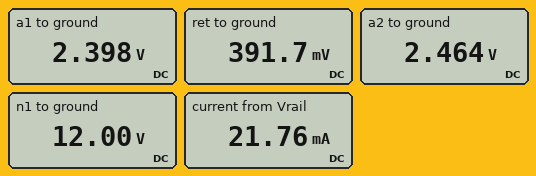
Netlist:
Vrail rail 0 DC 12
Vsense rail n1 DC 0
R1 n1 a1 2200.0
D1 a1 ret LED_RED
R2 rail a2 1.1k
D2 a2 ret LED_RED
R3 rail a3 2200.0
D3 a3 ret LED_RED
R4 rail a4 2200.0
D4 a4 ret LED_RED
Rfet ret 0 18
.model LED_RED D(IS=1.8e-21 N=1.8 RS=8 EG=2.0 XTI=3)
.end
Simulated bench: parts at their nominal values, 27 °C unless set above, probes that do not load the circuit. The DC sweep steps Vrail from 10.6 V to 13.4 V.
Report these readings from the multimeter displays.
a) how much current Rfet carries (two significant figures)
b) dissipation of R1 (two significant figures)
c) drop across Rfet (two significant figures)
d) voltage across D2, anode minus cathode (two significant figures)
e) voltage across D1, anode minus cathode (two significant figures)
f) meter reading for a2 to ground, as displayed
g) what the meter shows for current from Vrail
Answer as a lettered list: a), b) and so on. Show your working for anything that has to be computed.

a) (391.7 mV) / 18 Ω = 22 mA
b) (12 V - 2.398 V)^2 / 2.2 kΩ = 42 mW
c) 391.7 mV = 390 mV
d) 2.464 V - 391.7 mV = 2.1 V
e) 2.398 V - 391.7 mV = 2.0 V
f) 2.464 V
g) 21.76 mA
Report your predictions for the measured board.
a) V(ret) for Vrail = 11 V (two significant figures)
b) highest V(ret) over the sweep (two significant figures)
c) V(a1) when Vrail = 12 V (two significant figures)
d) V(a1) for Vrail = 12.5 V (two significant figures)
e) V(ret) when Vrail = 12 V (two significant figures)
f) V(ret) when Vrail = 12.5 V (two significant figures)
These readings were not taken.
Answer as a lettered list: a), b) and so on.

a) 350 mV
b) 450 mV
c) 2.4 V
d) 2.4 V
e) 390 mV
f) 410 mV
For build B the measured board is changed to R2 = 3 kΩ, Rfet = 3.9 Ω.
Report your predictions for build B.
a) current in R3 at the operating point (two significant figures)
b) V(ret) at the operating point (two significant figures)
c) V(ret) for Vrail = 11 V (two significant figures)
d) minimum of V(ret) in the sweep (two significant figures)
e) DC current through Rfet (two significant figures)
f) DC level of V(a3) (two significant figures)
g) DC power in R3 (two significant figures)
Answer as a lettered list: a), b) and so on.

a) 4.5 mA
b) 66 mV
c) 59 mV
d) 57 mV
e) 17 mA
f) 2.1 V
g) 45 mW
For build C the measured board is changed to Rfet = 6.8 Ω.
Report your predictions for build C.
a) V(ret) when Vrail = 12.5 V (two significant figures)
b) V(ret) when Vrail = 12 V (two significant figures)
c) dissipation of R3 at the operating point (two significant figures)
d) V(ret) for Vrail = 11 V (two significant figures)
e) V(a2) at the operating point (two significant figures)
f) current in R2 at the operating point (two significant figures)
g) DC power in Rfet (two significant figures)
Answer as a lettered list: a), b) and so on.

a) 160 mV
b) 150 mV
c) 44 mW
d) 140 mV
e) 2.2 V
f) 8.9 mA
g) 3.4 mW
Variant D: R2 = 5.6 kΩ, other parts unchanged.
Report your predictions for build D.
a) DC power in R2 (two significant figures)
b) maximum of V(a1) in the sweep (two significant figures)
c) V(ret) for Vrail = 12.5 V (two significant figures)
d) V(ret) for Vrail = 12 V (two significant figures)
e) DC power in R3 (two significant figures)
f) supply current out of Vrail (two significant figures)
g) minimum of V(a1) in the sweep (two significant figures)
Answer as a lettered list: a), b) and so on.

a) 17 mW
b) 2.3 V
c) 280 mV
d) 270 mV
e) 43 mW
f) 15 mA
g) 2.2 V
